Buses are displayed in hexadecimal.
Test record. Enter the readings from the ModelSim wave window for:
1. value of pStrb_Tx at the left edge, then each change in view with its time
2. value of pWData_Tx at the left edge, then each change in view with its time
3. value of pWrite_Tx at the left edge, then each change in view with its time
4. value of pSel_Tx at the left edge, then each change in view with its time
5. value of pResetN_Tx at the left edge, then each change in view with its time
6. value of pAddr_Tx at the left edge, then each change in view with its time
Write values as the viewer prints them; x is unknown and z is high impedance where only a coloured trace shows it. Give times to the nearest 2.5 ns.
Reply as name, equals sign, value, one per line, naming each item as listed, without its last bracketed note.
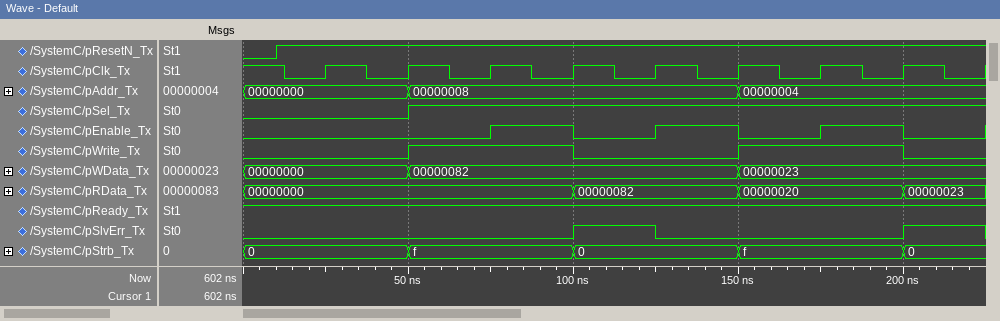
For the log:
value of pStrb_Tx at the left edge, then each change in view with its time = 0, f at 50 ns, 0 at 100 ns, f at 150 ns, 0 at 200 ns
value of pWData_Tx at the left edge, then each change in view with its time = 00000000, 00000082 at 50 ns, 00000023 at 150 ns
value of pWrite_Tx at the left edge, then each change in view with its time = 0, 1 at 50 ns, 0 at 100 ns, 1 at 150 ns, 0 at 200 ns
value of pSel_Tx at the left edge, then each change in view with its time = 0, 1 at 50 ns
value of pResetN_Tx at the left edge, then each change in view with its time = 0, 1 at 10 ns
value of pAddr_Tx at the left edge, then each change in view with its time = 00000000, 00000008 at 50 ns, 00000004 at 150 ns
